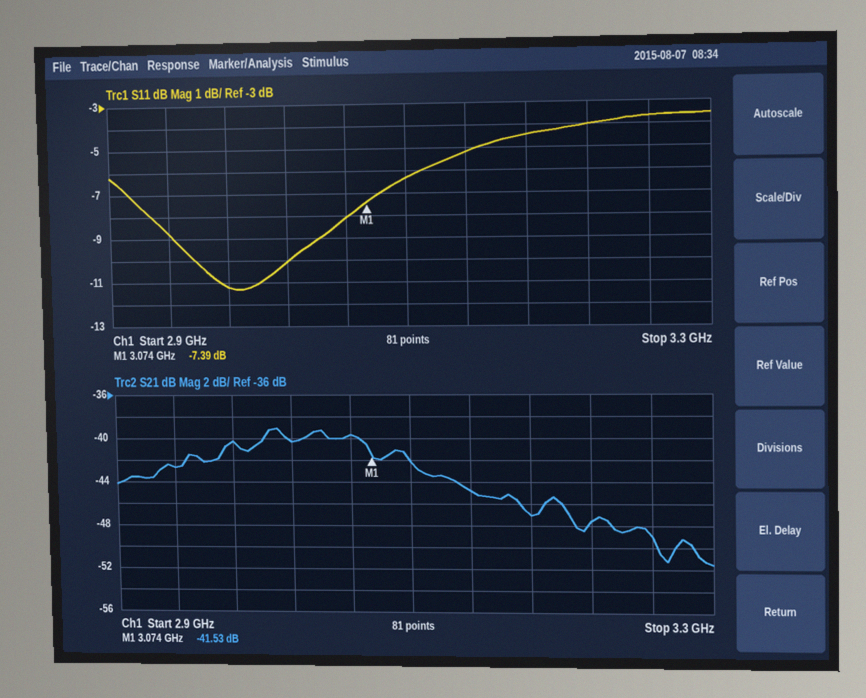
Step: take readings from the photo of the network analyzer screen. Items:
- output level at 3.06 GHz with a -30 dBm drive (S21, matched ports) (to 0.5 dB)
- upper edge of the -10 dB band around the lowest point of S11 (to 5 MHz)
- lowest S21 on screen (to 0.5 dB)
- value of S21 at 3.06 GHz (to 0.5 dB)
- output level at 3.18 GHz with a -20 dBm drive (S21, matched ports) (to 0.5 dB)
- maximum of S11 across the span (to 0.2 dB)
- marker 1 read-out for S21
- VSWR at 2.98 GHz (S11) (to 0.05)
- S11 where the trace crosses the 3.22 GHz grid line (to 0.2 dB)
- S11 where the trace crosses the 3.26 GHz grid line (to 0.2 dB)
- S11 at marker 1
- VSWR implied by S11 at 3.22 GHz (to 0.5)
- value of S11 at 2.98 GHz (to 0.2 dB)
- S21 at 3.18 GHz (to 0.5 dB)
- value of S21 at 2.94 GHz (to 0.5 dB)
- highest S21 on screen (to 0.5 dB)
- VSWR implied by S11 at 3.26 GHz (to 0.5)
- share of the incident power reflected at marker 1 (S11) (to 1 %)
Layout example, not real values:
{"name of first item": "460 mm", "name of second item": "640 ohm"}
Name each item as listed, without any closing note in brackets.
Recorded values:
{"output level at 3.06 GHz with a -30 dBm drive (S21, matched ports)": "-69.5 dBm", "upper edge of the -10 dB band around the lowest point of S11": "3.020 GHz", "lowest S21 on screen": "-51.5 dB", "value of S21 at 3.06 GHz": "-39.5 dB", "output level at 3.18 GHz with a -20 dBm drive (S21, matched ports)": "-67.0 dBm", "maximum of S11 across the span": "-3.6 dB", "marker 1 read-out for S21": "-41.53 dB", "VSWR at 2.98 GHz (S11)": "1.75", "S11 where the trace crosses the 3.22 GHz grid line": "-4.0 dB", "S11 where the trace crosses the 3.26 GHz grid line": "-3.6 dB", "S11 at marker 1": "-7.39 dB", "VSWR implied by S11 at 3.22 GHz": "4.5", "value of S11 at 2.98 GHz": "-11.2 dB", "S21 at 3.18 GHz": "-47.0 dB", "value of S21 at 2.94 GHz": "-42.5 dB", "highest S21 on screen": "-39.0 dB", "VSWR implied by S11 at 3.26 GHz": "5.0", "share of the incident power reflected at marker 1 (S11)": "18 %"}
